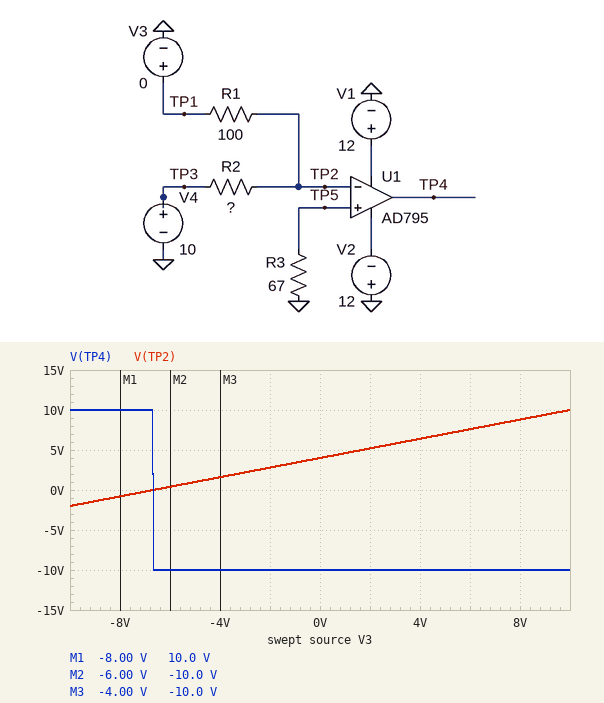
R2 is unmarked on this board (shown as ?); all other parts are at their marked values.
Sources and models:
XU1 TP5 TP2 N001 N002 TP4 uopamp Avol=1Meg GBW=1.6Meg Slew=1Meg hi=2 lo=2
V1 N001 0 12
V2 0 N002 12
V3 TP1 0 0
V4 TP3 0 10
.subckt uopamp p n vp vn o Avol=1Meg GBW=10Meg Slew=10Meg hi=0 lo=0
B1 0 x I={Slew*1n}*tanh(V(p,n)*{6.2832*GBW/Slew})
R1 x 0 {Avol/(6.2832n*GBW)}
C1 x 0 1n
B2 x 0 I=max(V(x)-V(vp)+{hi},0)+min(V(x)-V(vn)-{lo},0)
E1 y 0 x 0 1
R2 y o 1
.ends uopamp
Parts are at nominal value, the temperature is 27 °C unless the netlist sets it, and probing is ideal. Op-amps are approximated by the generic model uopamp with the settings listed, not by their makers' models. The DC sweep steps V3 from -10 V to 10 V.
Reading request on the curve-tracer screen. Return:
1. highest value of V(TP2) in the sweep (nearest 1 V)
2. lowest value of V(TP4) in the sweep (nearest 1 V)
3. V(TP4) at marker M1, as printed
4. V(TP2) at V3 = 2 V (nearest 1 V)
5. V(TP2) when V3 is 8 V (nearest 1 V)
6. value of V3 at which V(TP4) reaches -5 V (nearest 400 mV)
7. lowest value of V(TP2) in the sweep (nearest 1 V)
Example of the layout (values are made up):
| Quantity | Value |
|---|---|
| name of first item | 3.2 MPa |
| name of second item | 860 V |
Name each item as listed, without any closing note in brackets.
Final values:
| Quantity | Value |
|---|---|
| highest value of V(TP2) in the sweep | 10 V |
| lowest value of V(TP4) in the sweep | -10 V |
| V(TP4) at marker M1, as printed | 10.0 V |
| V(TP2) at V3 = 2 V | 5 V |
| V(TP2) when V3 is 8 V | 9 V |
| value of V3 at which V(TP4) reaches -5 V | -6.8 V |
| lowest value of V(TP2) in the sweep | -2 V |
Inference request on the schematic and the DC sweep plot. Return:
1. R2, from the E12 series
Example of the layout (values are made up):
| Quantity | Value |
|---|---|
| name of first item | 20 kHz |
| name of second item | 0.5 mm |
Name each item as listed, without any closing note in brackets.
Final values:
| Quantity | Value |
|---|---|
| R2, from the E12 series | 150 Ω |
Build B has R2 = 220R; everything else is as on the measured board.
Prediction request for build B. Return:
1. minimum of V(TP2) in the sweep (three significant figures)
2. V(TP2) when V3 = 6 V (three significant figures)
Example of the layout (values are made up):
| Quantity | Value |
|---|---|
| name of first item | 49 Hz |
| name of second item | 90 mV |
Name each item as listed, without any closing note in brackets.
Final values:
| Quantity | Value |
|---|---|
| minimum of V(TP2) in the sweep | -3.75 V |
| V(TP2) when V3 = 6 V | 7.25 V |
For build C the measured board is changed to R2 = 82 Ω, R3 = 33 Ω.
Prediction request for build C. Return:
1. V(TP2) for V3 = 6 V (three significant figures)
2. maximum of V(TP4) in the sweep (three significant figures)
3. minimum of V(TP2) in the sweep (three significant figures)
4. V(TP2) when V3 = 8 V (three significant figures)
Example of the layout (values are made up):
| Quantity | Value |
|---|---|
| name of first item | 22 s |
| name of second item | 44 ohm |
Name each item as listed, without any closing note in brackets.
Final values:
| Quantity | Value |
|---|---|
| V(TP2) for V3 = 6 V | 8.20 V |
| maximum of V(TP4) in the sweep | -10.0 V |
| minimum of V(TP2) in the sweep | 989 mV |
| V(TP2) when V3 = 8 V | 9.10 V |
